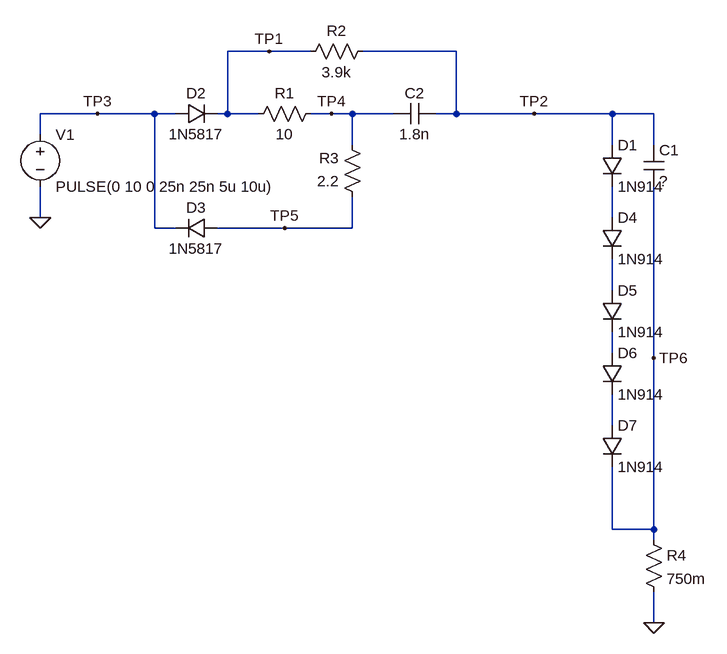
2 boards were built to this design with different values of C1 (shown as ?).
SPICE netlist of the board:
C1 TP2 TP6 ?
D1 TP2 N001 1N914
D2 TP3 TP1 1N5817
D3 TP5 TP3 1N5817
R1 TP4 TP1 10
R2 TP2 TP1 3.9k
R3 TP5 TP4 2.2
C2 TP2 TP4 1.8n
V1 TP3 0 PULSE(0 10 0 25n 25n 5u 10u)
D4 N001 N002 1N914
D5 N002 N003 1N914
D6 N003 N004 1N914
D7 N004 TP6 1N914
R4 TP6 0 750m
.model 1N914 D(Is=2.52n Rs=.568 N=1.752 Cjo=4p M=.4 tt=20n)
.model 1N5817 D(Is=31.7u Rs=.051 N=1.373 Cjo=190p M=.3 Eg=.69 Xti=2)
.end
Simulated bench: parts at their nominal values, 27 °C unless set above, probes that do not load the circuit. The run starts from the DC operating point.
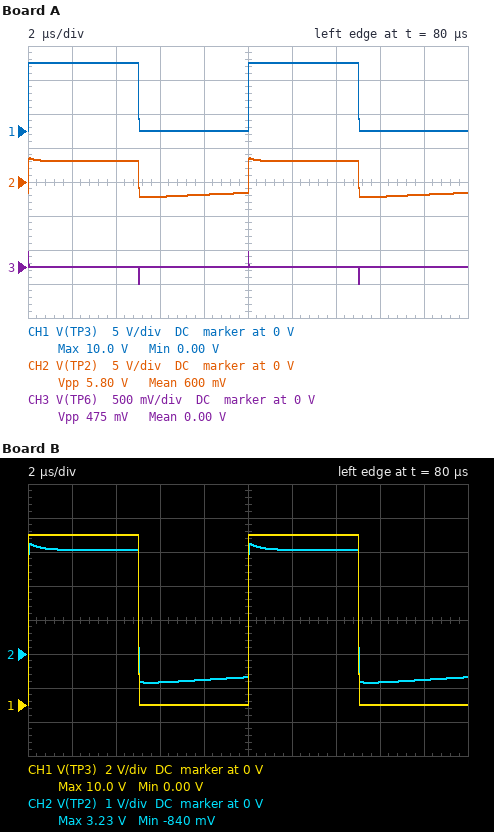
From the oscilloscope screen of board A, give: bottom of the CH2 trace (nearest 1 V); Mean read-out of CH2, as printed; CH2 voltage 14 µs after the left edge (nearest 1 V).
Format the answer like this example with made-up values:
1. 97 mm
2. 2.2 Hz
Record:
1. -2 V
2. 600 mV
3. 3 V
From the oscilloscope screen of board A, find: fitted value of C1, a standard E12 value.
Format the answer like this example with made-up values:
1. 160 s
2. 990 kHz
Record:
1. 1.5 nF
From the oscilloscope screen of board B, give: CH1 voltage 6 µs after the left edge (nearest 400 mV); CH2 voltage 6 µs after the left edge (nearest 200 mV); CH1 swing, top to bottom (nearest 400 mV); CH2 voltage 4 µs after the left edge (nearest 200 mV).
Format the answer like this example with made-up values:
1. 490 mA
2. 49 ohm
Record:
1. 0 V
2. -800 mV
3. 10.0 V
4. 3.0 V
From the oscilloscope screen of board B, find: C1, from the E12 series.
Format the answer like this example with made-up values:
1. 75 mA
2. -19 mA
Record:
1. 2.7 nF
